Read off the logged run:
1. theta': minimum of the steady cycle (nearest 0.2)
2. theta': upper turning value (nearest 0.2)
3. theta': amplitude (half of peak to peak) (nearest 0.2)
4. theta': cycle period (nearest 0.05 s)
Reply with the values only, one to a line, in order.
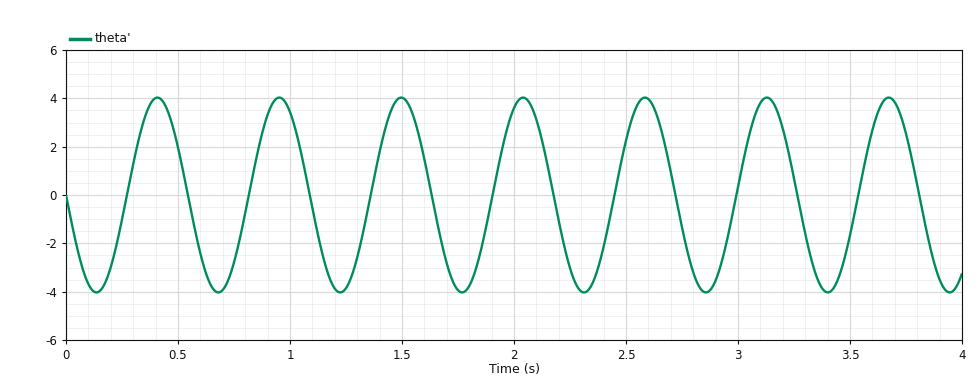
-4.0
4.0
4.0
0.55 s
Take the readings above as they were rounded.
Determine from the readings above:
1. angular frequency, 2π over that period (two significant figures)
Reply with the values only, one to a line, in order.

11 rad/s
